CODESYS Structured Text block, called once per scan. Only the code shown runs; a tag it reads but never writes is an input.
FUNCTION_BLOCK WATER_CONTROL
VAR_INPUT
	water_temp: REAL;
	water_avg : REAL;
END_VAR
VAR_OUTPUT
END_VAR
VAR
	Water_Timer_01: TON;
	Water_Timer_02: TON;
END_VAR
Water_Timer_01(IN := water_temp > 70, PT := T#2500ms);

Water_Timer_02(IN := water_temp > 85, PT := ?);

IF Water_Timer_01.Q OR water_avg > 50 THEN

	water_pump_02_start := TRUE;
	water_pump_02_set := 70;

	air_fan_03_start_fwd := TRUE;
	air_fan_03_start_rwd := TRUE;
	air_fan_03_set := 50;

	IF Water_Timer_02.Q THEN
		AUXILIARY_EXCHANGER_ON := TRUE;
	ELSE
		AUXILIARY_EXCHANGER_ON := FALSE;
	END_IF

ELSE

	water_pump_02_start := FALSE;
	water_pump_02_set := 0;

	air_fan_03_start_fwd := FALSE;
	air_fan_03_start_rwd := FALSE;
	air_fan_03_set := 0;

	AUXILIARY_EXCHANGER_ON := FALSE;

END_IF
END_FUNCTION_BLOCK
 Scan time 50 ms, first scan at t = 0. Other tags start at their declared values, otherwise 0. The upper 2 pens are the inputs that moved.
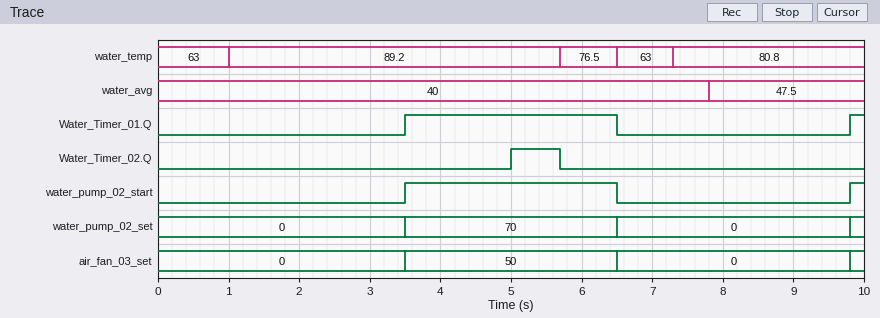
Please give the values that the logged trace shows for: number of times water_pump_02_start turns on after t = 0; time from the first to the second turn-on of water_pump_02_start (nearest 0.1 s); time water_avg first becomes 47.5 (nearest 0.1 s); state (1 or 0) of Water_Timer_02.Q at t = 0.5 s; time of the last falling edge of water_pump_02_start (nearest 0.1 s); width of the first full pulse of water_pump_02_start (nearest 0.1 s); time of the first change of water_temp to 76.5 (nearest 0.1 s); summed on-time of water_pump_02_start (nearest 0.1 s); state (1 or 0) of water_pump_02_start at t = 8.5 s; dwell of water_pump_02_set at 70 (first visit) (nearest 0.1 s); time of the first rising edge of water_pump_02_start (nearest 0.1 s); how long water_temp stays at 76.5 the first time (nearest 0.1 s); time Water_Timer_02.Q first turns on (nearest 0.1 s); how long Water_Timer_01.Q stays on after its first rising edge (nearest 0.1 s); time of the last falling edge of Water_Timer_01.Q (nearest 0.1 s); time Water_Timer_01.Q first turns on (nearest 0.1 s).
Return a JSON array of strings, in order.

["2", "6.3 s", "7.8 s", "0", "6.5 s", "3.0 s", "5.7 s", "3.2 s", "0", "3.0 s", "3.5 s", "0.8 s", "5.0 s", "3.0 s", "6.5 s", "3.5 s"]
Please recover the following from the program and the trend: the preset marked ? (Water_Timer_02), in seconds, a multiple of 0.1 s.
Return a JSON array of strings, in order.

["4.0 s"]
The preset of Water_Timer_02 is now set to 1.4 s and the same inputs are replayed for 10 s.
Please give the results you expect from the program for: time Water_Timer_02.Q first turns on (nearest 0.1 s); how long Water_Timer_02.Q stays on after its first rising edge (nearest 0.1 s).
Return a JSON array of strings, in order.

["2.4 s", "3.3 s"]
